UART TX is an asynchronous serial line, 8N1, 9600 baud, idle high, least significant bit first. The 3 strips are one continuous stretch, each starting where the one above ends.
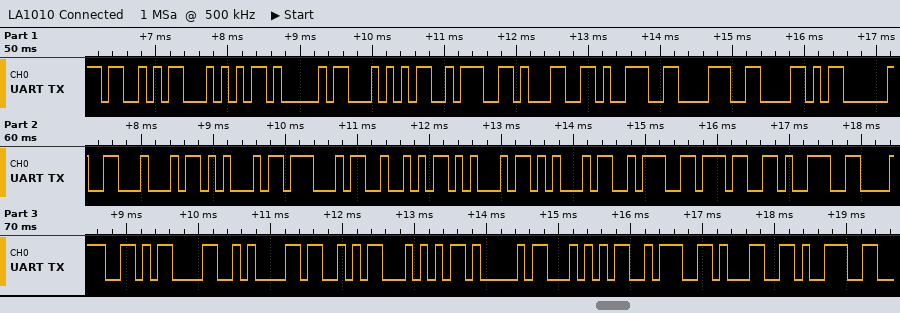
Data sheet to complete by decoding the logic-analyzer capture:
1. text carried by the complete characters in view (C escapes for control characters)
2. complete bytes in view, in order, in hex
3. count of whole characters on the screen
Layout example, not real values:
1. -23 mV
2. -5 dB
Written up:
1. "STAT:198X DEGREE:798\r\nSTAT:19"
2. 0x53 0x54 0x41 0x54 0x3A 0x31 0x39 0x38 0x58 0x20 0x44 0x45 0x47 0x52 0x45 0x45 0x3A 0x37 0x39 0x38 0x0D 0x0A 0x53 0x54 0x41 0x54 0x3A 0x31 0x39
3. 29
